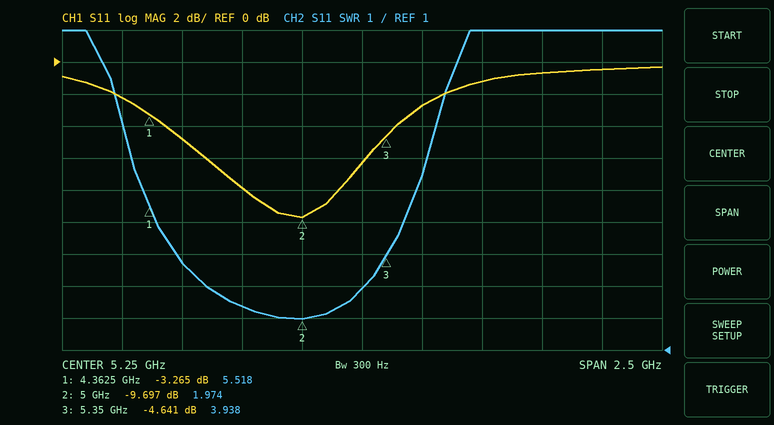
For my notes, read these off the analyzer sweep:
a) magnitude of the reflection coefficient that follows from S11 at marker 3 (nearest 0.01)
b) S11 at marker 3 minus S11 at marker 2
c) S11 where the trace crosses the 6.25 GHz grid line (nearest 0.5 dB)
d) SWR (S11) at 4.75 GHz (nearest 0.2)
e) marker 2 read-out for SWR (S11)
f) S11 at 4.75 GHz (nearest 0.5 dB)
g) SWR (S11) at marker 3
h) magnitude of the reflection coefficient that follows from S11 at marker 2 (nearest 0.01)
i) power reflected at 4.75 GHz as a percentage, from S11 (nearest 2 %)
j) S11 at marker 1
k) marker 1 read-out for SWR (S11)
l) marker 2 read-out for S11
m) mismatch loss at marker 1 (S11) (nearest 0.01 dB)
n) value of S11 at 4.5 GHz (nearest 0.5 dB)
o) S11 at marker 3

0.59
5.056 dB
-0.5 dB
2.4
1.974
-8.0 dB
3.938
0.33
16 %
-3.265 dB
5.518
-9.697 dB
2.77 dB
-5.0 dB
-4.641 dB
